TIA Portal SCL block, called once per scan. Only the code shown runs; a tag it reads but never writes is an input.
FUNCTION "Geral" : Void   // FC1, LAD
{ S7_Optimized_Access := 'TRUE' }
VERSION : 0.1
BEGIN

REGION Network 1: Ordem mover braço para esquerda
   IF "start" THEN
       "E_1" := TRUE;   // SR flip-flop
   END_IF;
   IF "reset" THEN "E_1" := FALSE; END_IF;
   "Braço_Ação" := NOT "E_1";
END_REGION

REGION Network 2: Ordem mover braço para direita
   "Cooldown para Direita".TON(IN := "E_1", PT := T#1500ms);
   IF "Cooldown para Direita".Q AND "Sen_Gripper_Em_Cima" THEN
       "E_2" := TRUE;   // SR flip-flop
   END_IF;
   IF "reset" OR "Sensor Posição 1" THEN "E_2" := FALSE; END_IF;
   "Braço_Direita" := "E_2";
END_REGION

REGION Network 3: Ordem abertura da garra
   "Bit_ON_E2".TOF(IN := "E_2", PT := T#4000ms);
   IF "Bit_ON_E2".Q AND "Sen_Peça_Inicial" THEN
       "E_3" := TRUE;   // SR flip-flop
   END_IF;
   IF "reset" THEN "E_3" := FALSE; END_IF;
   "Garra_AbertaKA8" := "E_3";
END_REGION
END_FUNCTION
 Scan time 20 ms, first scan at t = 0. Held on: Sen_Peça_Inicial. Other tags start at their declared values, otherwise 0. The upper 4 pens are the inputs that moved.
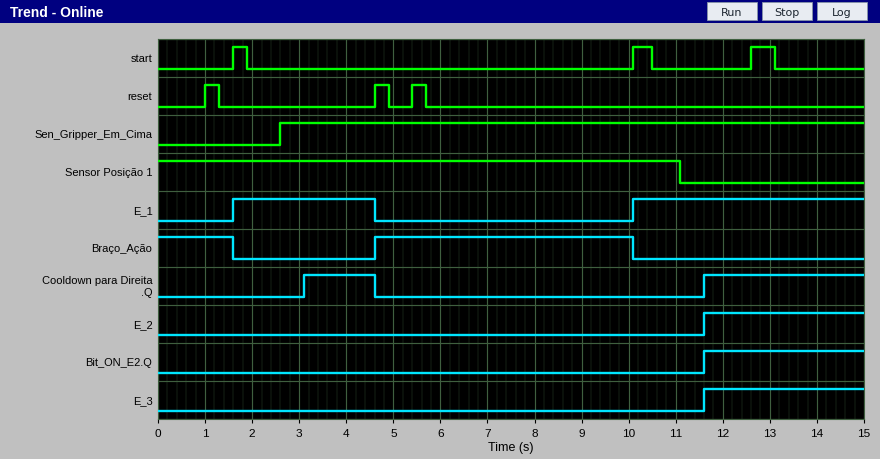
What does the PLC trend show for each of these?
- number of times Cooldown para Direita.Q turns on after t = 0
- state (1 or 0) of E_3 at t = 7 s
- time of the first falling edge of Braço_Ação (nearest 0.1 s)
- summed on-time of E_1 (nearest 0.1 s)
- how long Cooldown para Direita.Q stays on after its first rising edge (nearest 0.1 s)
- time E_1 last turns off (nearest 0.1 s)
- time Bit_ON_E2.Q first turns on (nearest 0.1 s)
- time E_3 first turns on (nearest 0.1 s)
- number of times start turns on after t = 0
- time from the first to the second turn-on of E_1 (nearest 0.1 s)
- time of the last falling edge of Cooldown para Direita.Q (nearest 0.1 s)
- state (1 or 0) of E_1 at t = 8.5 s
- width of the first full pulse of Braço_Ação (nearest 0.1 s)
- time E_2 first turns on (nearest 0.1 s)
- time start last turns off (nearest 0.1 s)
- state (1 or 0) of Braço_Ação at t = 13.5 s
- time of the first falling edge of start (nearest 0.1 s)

2
0
1.6 s
7.9 s
1.5 s
4.6 s
11.6 s
11.6 s
3
8.5 s
4.6 s
0
5.5 s
11.6 s
13.1 s
0
1.9 s
